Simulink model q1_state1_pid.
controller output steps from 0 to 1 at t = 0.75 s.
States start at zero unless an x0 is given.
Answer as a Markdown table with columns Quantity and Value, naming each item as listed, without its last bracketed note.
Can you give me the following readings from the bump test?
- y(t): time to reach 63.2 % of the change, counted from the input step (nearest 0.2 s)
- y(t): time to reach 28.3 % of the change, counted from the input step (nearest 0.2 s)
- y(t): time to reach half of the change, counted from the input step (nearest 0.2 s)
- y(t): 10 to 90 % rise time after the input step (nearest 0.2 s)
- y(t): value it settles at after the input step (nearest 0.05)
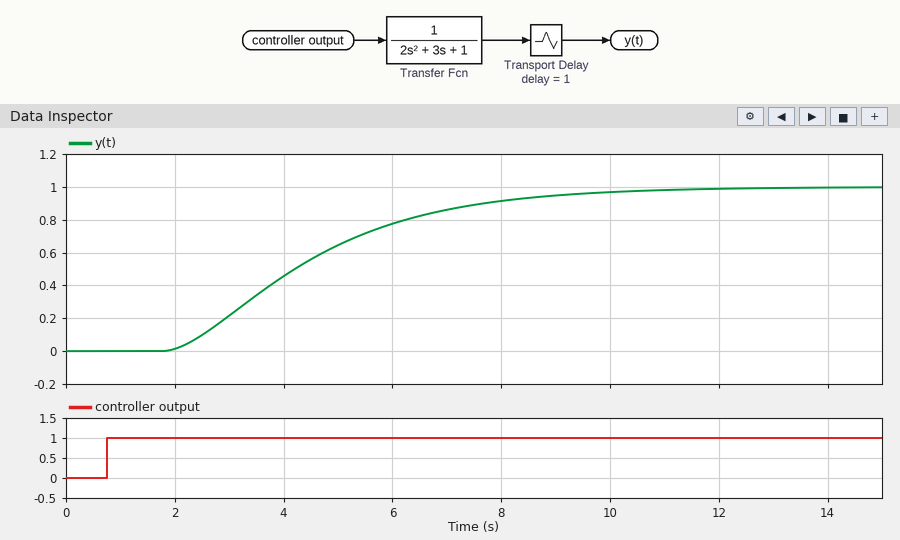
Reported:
| Quantity | Value |
|---|---|
| y(t): time to reach 63.2 % of the change, counted from the input step | 4.2 s |
| y(t): time to reach 28.3 % of the change, counted from the input step | 2.6 s |
| y(t): time to reach half of the change, counted from the input step | 3.4 s |
| y(t): 10 to 90 % rise time after the input step | 5.2 s |
| y(t): value it settles at after the input step | 1.00 |
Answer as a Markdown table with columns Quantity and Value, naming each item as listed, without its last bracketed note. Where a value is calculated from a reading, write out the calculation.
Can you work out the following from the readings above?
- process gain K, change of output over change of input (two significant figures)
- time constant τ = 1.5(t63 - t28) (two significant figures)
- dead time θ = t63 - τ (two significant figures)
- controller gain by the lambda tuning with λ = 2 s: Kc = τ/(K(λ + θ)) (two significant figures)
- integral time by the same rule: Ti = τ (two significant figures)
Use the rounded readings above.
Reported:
| Quantity | Value |
|---|---|
| process gain K, change of output over change of input | (1 - 0) / 1 = 1.0 |
| time constant τ = 1.5(t63 - t28) | 1.5 × (4.2 - 2.6) = 2.4 s |
| dead time θ = t63 - τ | 4.2 - 2.4 = 1.8 s |
| controller gain by the lambda tuning with λ = 2 s: Kc = τ/(K(λ + θ)) | 2.4 / (1 × (2 + 1.8)) = 0.63 |
| integral time by the same rule: Ti = τ | 2.4 s |
